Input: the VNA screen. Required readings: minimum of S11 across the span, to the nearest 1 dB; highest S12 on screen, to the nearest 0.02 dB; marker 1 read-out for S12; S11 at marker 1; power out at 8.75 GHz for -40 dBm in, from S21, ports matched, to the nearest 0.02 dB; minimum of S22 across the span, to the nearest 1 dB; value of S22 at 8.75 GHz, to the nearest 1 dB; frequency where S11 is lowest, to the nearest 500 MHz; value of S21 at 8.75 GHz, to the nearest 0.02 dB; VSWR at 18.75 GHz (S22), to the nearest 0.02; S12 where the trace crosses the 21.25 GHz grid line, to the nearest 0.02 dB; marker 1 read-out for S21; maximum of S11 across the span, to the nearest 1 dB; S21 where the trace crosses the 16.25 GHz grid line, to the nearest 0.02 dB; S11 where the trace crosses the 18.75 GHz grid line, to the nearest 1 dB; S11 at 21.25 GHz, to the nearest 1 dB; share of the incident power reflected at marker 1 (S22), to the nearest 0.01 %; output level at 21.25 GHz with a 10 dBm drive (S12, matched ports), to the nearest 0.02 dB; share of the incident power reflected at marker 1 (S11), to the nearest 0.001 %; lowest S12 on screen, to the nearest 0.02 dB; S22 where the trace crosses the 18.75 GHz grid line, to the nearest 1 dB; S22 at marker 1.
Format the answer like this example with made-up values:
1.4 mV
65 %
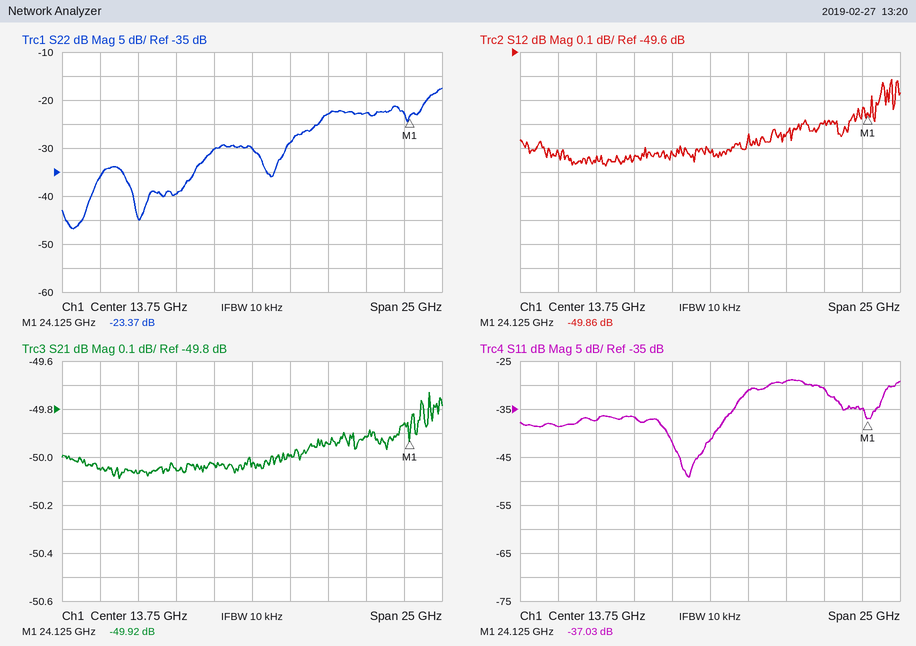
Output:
-49 dB
-49.72 dB
-49.86 dB
-37.03 dB
-90.06 dBm
-47 dB
-40 dB
12.5 GHz
-50.06 dB
1.16
-49.90 dB
-49.92 dB
-29 dB
-50.00 dB
-29 dB
-31 dB
0.46 %
-39.90 dBm
0.020 %
-50.08 dB
-23 dB
-23.37 dB
